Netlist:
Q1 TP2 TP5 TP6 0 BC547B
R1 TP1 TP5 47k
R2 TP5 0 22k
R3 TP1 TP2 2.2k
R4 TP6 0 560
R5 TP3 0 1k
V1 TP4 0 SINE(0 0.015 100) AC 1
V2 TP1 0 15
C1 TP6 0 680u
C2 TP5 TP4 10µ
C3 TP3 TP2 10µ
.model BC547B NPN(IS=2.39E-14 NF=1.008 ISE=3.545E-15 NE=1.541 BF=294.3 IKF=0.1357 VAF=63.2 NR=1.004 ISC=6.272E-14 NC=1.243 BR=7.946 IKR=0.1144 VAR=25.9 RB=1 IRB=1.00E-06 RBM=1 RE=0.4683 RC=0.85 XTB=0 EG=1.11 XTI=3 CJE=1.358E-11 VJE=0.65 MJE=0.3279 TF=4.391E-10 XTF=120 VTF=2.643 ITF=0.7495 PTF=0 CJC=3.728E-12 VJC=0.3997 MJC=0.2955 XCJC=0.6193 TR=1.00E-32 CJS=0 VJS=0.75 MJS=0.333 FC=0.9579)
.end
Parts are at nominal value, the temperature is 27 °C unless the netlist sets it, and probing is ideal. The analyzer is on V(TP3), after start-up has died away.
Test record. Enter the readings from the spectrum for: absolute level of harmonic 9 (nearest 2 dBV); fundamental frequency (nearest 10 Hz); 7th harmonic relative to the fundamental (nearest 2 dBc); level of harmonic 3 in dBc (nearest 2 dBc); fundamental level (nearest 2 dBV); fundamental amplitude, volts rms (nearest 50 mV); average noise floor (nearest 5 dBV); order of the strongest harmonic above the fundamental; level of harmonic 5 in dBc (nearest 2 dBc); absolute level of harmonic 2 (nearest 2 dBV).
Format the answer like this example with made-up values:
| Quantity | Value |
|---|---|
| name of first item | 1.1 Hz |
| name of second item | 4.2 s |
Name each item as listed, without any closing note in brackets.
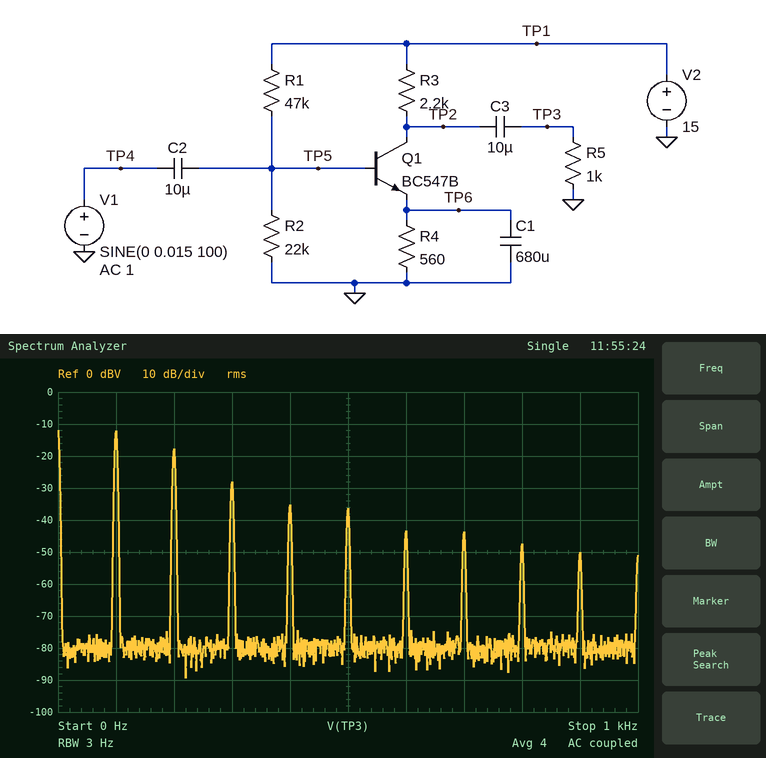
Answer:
| Quantity | Value |
|---|---|
| absolute level of harmonic 9 | -50 dBV |
| fundamental frequency | 100 Hz |
| 7th harmonic relative to the fundamental | -32 dBc |
| level of harmonic 3 in dBc | -16 dBc |
| fundamental level | -12 dBV |
| fundamental amplitude, volts rms | 250 mV |
| average noise floor | -80 dBV |
| order of the strongest harmonic above the fundamental | 2 |
| level of harmonic 5 in dBc | -24 dBc |
| absolute level of harmonic 2 | -18 dBV |
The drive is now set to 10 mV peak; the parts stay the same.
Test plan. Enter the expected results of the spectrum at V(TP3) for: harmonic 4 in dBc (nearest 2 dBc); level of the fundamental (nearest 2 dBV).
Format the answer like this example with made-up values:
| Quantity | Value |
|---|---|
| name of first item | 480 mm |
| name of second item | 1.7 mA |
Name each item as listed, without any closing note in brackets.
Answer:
| Quantity | Value |
|---|---|
| harmonic 4 in dBc | -18 dBc |
| level of the fundamental | -26 dBV |
